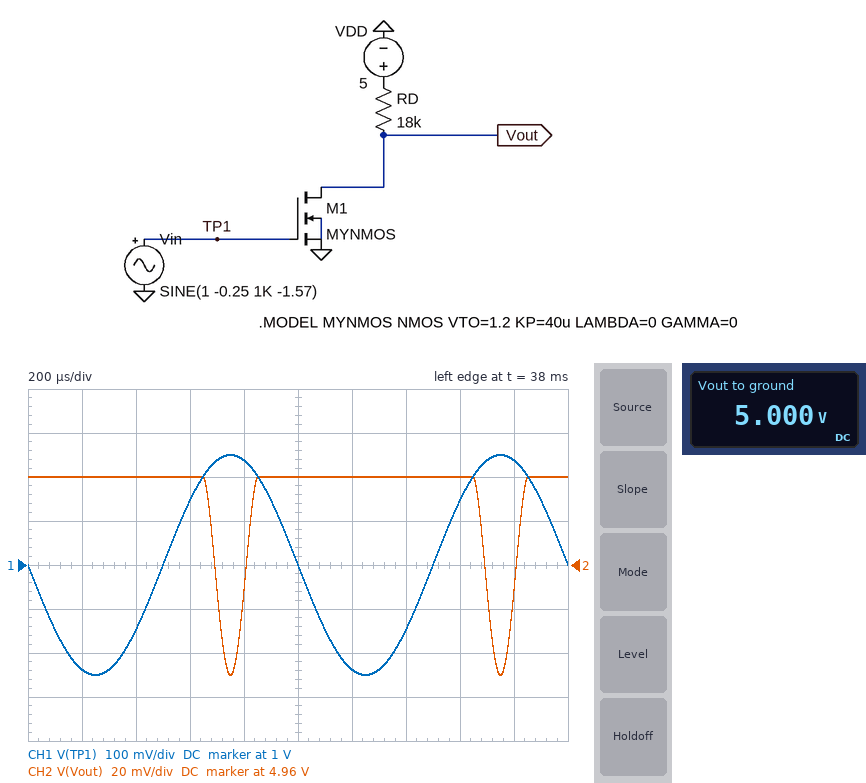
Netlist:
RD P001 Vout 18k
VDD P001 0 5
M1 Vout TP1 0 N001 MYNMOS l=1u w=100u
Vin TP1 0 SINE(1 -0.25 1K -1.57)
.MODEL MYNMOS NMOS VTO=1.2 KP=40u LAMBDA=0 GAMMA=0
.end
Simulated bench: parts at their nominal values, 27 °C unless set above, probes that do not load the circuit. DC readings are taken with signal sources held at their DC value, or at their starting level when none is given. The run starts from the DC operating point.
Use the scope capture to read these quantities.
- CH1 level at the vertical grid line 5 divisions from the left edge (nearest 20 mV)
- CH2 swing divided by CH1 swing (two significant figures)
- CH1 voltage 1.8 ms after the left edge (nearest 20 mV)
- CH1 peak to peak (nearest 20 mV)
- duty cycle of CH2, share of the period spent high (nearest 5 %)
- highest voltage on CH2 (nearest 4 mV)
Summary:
1.00 V
0.18
1.24 V
500 mV
90 %
5.000 V
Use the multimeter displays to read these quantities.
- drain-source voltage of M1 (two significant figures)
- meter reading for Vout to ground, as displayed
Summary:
5.0 V
5.000 V
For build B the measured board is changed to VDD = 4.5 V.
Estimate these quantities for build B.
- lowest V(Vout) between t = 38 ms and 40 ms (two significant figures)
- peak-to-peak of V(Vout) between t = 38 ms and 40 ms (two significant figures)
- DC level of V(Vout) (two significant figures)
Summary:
4.4 V
90 mV
4.5 V
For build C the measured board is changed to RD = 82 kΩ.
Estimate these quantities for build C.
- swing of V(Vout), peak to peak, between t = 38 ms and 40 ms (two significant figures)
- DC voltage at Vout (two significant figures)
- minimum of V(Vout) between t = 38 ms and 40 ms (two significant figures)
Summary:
410 mV
5.0 V
4.6 V
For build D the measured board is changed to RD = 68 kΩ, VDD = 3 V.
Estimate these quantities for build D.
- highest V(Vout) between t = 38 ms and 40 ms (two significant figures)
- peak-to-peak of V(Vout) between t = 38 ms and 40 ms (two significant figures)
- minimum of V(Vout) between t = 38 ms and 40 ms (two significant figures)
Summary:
3.0 V
340 mV
2.7 V
